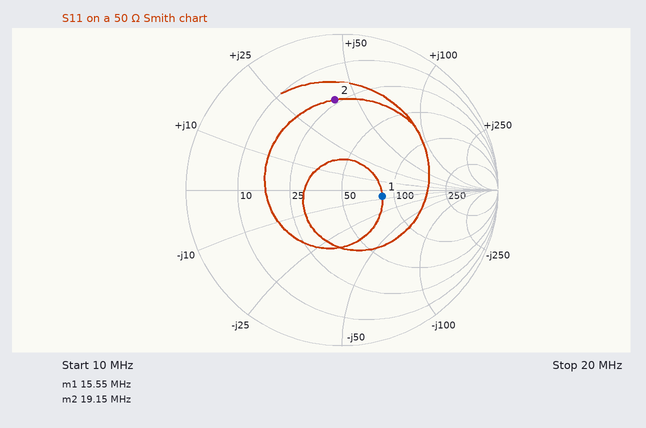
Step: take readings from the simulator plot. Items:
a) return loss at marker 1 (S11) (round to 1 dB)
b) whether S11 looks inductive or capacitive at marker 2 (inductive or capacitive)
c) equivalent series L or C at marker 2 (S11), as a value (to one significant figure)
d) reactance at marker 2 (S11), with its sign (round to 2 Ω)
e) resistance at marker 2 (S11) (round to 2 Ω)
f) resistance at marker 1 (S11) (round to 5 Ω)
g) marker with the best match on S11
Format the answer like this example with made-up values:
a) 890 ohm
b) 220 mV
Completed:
a) 12 dB
b) inductive
c) 300 nH
d) +40 Ω
e) 24 Ω
f) 85 Ω
g) marker 1
